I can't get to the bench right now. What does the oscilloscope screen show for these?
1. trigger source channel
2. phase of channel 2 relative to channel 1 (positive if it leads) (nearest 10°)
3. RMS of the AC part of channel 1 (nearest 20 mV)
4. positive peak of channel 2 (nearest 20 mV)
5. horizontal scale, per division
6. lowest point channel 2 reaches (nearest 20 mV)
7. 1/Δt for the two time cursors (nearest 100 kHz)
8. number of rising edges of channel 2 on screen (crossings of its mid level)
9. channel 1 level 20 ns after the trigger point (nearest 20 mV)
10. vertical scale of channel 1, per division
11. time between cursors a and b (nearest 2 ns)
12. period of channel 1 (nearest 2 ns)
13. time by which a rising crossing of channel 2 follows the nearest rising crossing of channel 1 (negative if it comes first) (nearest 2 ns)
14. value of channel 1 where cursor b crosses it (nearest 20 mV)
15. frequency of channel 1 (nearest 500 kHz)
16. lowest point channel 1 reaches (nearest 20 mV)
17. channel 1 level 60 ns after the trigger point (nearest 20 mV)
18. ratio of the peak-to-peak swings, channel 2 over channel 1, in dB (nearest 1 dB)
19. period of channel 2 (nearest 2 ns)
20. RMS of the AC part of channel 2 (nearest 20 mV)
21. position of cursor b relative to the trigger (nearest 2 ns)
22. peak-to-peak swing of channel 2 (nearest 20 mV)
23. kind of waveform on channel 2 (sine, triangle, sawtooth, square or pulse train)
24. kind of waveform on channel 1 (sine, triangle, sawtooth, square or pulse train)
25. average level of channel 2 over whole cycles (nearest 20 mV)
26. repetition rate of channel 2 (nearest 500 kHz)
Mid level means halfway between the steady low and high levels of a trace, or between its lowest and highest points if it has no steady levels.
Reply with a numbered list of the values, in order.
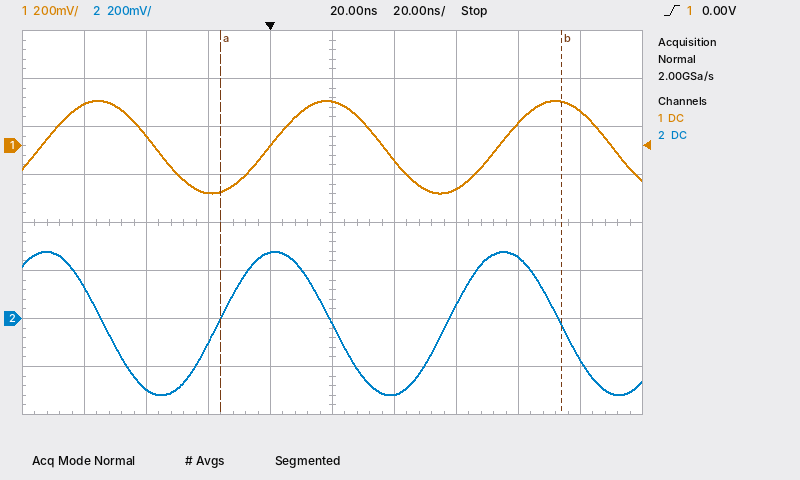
1. channel 1
2. +80°
3. 140 mV
4. 280 mV
5. 20 ns
6. -320 mV
7. 9.1 MHz
8. 2
9. 180 mV
10. 200 mV
11. 110 ns
12. 74 ns
13. -16 ns
14. 180 mV
15. 13.5 MHz
16. -200 mV
17. -180 mV
18. 4 dB
19. 74 ns
20. 220 mV
21. +94 ns
22. 600 mV
23. sine
24. sine
25. -20 mV
26. 13.5 MHz
